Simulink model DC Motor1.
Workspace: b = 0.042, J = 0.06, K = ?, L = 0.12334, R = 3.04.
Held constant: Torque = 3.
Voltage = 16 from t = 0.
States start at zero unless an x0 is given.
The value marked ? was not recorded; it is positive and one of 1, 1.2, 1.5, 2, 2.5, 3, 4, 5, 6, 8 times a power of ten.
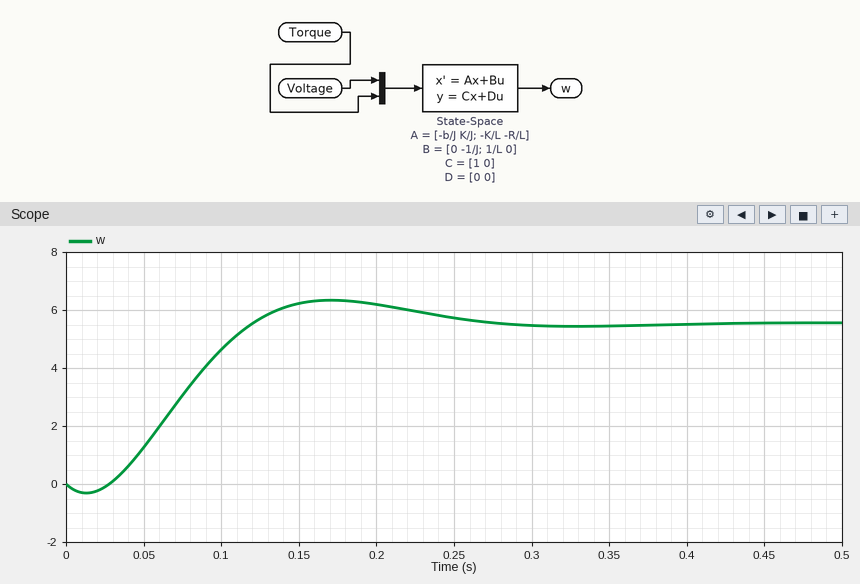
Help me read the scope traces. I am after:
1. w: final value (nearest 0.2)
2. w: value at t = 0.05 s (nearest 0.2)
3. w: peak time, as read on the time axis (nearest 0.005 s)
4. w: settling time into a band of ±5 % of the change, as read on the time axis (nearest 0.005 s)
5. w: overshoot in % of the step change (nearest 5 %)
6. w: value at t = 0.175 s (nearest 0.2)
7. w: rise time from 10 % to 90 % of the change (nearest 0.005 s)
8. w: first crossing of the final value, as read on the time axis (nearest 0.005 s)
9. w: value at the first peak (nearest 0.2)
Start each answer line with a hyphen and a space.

- 5.6
- 1.2
- 0.170 s
- 0.240 s
- 15 %
- 6.4
- 0.070 s
- 0.120 s
- 6.4
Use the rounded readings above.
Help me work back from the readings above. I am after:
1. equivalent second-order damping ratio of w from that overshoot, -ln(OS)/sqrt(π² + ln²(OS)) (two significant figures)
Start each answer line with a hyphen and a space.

- 0.52
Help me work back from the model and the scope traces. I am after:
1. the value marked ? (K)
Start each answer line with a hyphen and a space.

- 2
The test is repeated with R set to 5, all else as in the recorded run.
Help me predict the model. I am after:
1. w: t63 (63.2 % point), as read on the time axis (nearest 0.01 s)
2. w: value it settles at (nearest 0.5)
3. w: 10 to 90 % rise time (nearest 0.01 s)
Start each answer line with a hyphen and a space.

- 0.10 s
- 4.0
- 0.11 s
